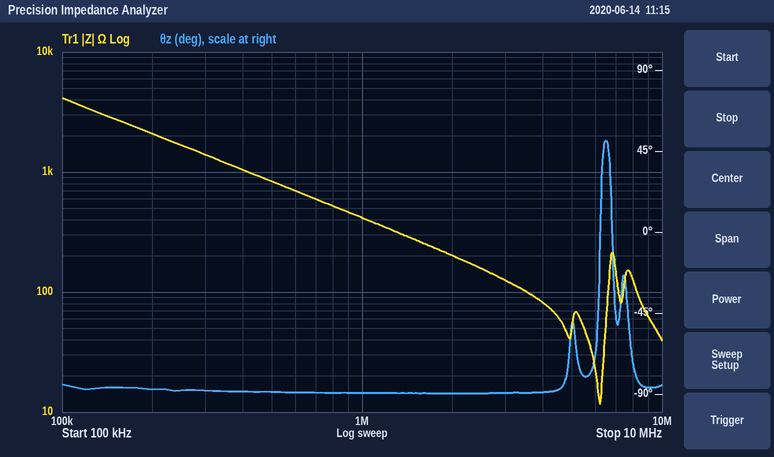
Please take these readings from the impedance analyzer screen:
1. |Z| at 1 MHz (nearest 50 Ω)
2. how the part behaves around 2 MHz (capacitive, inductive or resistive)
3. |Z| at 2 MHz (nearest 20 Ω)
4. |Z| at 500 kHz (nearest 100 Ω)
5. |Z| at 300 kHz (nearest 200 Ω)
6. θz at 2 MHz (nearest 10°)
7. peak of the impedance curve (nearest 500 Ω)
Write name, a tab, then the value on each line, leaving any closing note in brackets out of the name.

|Z| at 1 MHz	400 Ω
how the part behaves around 2 MHz	capacitive
|Z| at 2 MHz	200 Ω
|Z| at 500 kHz	800 Ω
|Z| at 300 kHz	1.4 kΩ
θz at 2 MHz	-90°
peak of the impedance curve	4.0 kΩ
